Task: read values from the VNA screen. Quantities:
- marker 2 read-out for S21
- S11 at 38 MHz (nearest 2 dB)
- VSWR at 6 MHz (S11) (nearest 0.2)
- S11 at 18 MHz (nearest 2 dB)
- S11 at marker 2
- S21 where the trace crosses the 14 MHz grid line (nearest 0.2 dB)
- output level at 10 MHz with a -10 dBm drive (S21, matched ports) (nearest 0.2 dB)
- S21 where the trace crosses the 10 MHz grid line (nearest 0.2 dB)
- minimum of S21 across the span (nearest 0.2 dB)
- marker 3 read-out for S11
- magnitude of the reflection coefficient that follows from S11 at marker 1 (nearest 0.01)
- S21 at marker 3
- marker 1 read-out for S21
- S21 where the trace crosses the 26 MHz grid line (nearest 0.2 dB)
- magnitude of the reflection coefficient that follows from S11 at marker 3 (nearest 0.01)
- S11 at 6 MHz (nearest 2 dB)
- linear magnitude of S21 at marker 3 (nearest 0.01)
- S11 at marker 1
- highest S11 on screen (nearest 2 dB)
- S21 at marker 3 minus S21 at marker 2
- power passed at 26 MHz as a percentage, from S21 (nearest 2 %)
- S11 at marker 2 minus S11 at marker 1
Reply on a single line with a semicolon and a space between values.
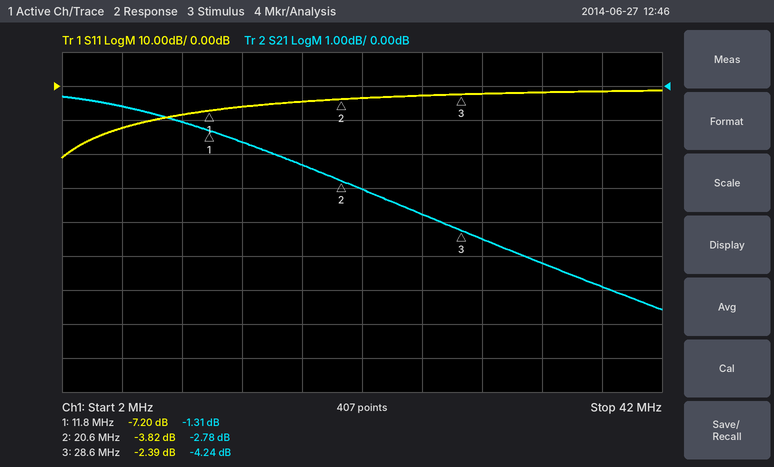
-2.78 dB; -2 dB; 1.6; -4 dB; -3.82 dB; -1.6 dB; -11.0 dBm; -1.0 dB; -6.6 dB; -2.39 dB; 0.44; -4.24 dB; -1.31 dB; -3.8 dB; 0.76; -12 dB; 0.61; -7.20 dB; -2 dB; -1.46 dB; 42 %; 3.38 dB
